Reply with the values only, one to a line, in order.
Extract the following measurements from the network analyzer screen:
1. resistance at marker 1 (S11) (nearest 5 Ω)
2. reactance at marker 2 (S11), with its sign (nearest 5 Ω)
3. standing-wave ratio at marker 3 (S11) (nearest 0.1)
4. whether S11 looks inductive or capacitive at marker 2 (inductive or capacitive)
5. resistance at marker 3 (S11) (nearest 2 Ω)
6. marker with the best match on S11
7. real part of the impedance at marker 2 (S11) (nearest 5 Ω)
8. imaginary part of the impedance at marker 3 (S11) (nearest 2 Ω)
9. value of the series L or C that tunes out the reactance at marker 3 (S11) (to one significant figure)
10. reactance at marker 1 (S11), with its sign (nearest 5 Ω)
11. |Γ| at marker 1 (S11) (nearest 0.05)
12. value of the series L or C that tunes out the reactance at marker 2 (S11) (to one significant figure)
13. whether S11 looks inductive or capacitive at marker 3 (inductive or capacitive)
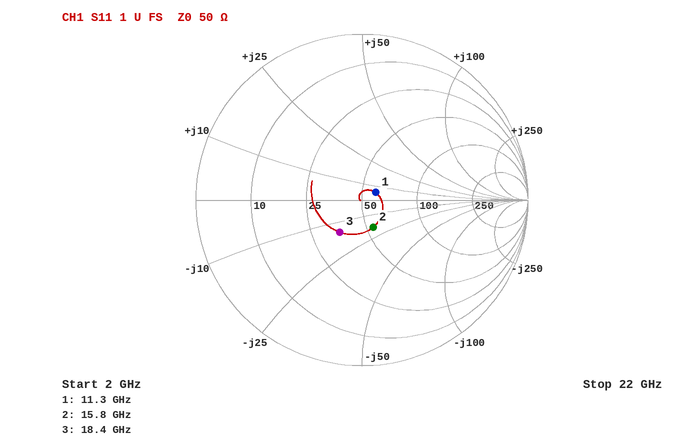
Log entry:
60 Ω
-20 Ω
1.6
capacitive
36 Ω
marker 1
55 Ω
-14 Ω
100 pH
+5 Ω
0.10
200 pH
capacitive
